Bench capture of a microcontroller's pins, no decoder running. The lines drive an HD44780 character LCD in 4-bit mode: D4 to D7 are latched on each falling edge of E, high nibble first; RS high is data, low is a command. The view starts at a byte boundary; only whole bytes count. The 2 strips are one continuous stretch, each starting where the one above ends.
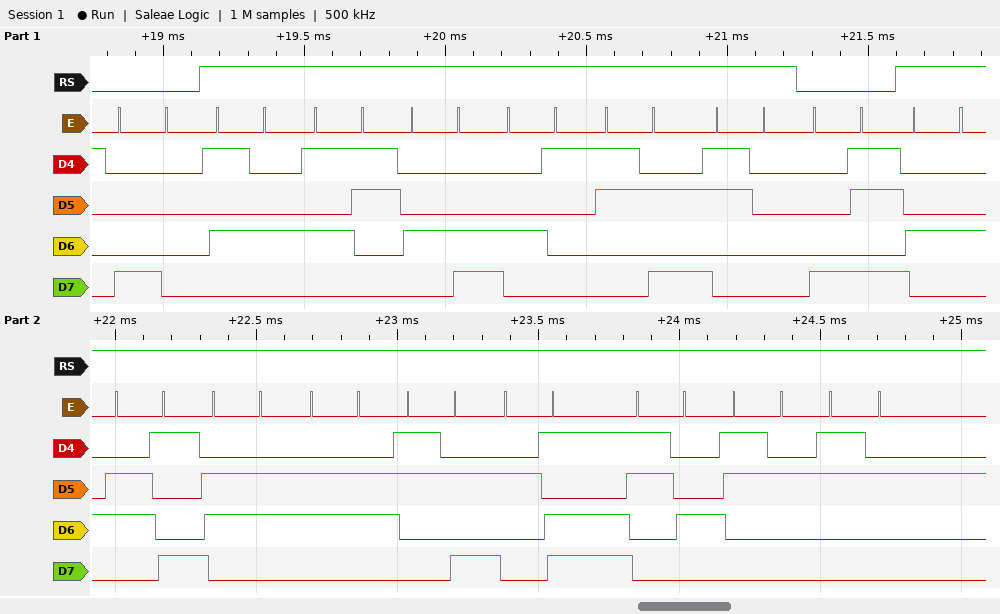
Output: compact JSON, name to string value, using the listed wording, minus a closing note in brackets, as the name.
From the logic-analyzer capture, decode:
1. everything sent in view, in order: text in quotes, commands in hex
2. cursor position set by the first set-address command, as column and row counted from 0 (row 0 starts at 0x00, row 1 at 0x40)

{"everything sent in view, in order: text in quotes, commands in hex": "0x80 \"TSLA:0\" 0x8B \"Diff:-422\"", "cursor position set by the first set-address command, as column and row counted from 0": "column 0, row 0"}
